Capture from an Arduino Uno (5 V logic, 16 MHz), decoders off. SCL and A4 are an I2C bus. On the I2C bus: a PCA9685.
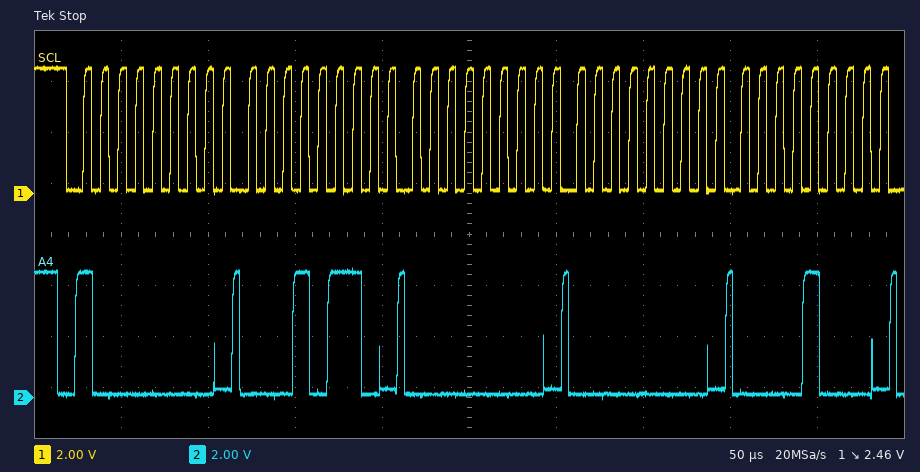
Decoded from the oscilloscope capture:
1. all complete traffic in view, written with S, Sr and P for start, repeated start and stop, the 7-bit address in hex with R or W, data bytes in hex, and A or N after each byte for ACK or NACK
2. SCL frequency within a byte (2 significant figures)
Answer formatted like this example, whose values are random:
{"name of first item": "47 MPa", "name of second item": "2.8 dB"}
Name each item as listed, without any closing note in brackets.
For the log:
{"all complete traffic in view, written with S, Sr and P for start, repeated start and stop, the 7-bit address in hex with R or W, data bytes in hex, and A or N after each byte for ACK or NACK": "S 40W A 16 A 00 A 00 A 08 A", "SCL frequency within a byte": "100 kHz"}
